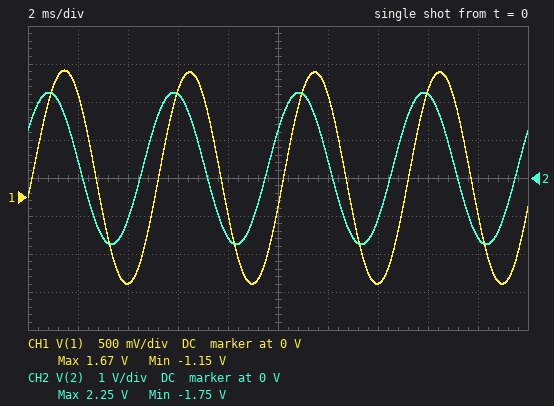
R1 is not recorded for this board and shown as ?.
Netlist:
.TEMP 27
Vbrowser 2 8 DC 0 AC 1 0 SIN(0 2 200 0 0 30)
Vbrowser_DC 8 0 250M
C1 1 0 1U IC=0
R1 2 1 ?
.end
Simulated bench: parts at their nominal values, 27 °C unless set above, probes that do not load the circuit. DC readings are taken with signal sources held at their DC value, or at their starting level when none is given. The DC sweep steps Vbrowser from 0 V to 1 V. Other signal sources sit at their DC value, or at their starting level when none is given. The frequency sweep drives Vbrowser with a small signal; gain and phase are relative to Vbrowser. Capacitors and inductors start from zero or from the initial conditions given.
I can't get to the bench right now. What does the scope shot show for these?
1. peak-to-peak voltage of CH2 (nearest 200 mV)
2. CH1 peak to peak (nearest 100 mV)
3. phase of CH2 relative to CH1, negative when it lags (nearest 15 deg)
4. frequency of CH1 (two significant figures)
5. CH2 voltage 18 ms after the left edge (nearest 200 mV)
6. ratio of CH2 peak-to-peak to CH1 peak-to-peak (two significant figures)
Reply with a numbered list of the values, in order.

1. 4.0 V
2. 2.8 V
3. 45 deg
4. 200 Hz
5. -1.6 V
6. 1.4
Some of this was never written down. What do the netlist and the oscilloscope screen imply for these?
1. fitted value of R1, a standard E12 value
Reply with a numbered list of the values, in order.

1. 820 Ω
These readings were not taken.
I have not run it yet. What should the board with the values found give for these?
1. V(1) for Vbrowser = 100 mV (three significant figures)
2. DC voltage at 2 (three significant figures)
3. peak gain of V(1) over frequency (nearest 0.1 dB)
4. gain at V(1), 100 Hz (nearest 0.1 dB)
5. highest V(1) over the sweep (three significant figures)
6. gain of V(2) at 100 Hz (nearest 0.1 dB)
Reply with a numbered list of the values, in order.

1. 350 mV
2. 250 mV
3. 0 dB
4. -1.0 dB
5. 1.25 V
6. 0 dB
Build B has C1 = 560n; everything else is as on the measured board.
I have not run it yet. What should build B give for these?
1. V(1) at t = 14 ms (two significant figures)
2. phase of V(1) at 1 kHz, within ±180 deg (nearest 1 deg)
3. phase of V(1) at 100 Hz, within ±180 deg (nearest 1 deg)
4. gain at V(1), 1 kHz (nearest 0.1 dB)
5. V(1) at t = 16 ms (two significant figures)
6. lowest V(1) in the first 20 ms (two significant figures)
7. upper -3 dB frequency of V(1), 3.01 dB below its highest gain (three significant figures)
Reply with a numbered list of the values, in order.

1. -1.4 V
2. -71 deg
3. -16 deg
4. -9.7 dB
5. 1.9 V
6. -1.5 V
7. 347 Hz
